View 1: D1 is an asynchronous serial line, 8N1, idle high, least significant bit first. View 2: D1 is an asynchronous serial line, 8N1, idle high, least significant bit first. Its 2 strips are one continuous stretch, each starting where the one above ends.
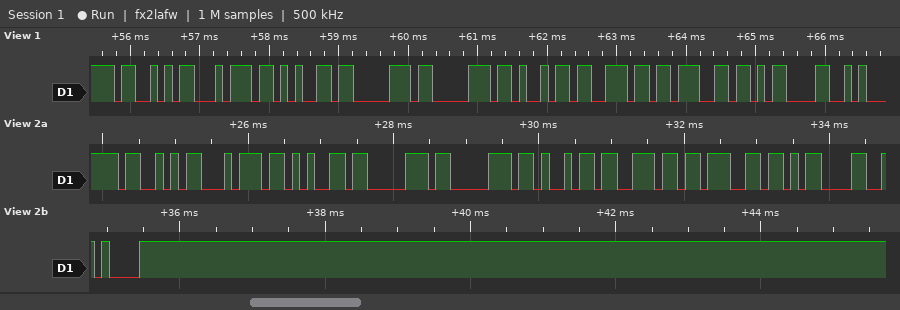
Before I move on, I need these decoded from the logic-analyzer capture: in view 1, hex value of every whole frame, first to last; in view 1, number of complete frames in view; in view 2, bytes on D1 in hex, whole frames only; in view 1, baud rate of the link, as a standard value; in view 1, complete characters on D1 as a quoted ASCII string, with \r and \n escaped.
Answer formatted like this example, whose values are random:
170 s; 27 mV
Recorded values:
53 74 65 70 70 69 6E 67 0D; 9; 53 74 65 70 70 69 6E 67 0D 0A; 9600 baud; "Stepping\r"
